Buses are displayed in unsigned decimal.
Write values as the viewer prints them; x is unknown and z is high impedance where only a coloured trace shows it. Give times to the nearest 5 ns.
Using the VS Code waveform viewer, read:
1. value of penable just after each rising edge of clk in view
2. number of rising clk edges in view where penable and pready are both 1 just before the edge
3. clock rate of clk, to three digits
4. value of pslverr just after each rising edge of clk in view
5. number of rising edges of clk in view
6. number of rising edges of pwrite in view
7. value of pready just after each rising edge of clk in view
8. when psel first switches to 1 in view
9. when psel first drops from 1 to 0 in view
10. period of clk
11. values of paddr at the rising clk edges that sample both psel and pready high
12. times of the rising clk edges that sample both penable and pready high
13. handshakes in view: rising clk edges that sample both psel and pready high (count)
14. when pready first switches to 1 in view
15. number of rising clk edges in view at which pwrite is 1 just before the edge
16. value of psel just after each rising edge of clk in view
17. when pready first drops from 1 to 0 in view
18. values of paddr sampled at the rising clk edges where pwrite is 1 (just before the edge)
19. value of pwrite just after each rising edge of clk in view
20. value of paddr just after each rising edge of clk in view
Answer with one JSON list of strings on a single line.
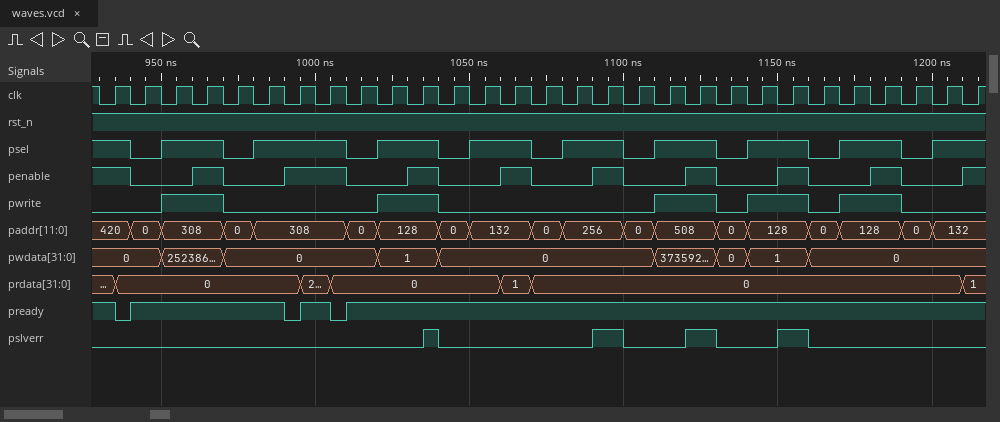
["1 0 0 1 0 0 1 1 0 0 1 0 0 1 0 0 1 0 0 1 0 0 1 0 0 1 0 0 1", "10", "100 MHz", "0 0 0 0 0 0 0 0 0 0 1 0 0 0 0 0 1 0 0 1 0 0 1 0 0 0 0 0 0", "29", "5", "0 1 1 1 1 1 1 0 1 1 1 1 1 1 1 1 1 1 1 1 1 1 1 1 1 1 1 1 1", "950 ns", "940 ns", "10 ns", "420, 308, 308, 308, 308, 128, 128, 132, 132, 256, 256, 508, 508, 128, 128, 128, 128, 132, 132", "935 ns, 965 ns, 1005 ns, 1035 ns, 1065 ns, 1095 ns, 1125 ns, 1155 ns, 1185 ns, 1215 ns", "19", "940 ns", "10", "1 0 1 1 0 1 1 1 0 1 1 0 1 1 0 1 1 0 1 1 0 1 1 0 1 1 0 1 1", "935 ns", "308, 308, 128, 128, 508, 508, 128, 128, 128, 128", "0 0 1 1 0 0 0 0 0 1 1 0 0 0 0 0 0 0 1 1 0 1 1 0 1 1 0 0 0", "420, 0, 308, 308, 0, 308, 308, 308, 0, 128, 128, 0, 132, 132, 0, 256, 256, 0, 508, 508, 0, 128, 128, 0, 128, 128, 0, 132, 132"]
